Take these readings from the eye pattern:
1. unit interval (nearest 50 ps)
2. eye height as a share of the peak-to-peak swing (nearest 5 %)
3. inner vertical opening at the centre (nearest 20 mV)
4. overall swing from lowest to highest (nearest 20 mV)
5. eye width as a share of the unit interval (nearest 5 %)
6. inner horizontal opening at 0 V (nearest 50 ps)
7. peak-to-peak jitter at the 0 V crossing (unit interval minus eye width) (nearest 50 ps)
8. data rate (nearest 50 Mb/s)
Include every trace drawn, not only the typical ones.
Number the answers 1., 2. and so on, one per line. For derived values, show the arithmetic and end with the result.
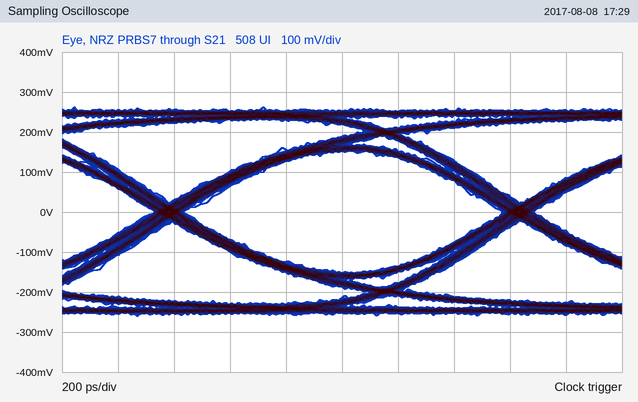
1. 1.25 ns
2. 300 mV / 520 mV ≈ 57.7 %, so 60 % to the nearest 5 %
3. 300 mV
4. 520 mV
5. 1.15 ns / 1.25 ns ≈ 92.0 %, so 90 % to the nearest 5 %
6. 1.15 ns
7. 100 ps
8. 800 Mb/s
